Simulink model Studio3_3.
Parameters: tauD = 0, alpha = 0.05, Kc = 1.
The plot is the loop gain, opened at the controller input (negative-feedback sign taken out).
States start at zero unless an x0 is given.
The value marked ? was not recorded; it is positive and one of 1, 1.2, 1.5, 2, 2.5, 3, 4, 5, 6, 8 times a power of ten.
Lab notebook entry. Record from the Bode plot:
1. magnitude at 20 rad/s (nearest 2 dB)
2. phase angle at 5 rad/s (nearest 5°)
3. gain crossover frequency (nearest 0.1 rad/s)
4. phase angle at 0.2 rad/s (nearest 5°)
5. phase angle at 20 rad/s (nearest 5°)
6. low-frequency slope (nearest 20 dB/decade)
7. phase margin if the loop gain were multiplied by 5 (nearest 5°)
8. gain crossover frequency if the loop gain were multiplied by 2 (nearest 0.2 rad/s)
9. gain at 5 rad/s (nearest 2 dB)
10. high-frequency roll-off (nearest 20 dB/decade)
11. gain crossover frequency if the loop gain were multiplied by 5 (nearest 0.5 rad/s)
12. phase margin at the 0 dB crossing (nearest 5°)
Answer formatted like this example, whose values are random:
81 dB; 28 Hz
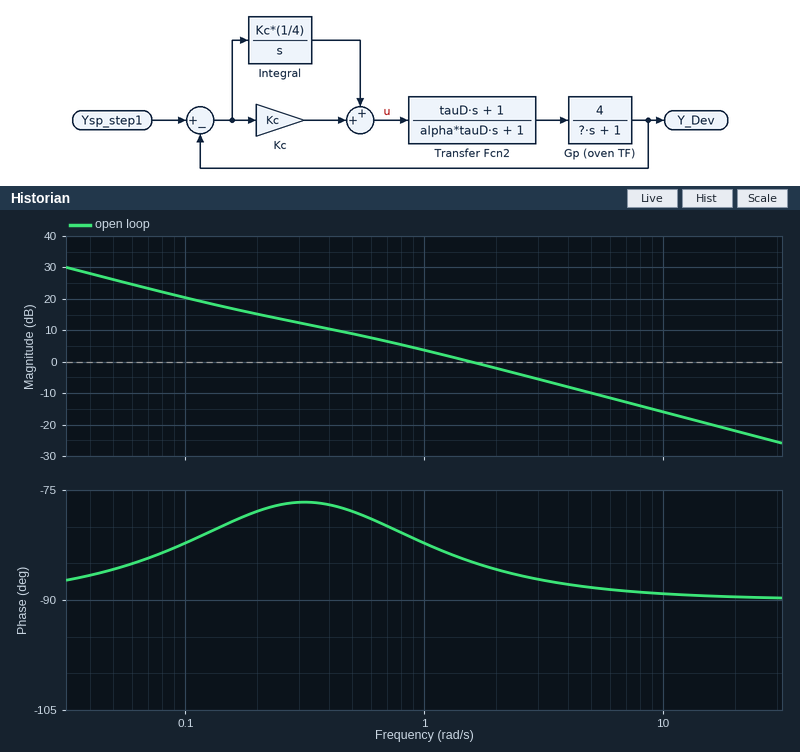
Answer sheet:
-22 dB; -90°; 1.6 rad/s; -80°; -90°; -20 dB/decade; 90°; 3.2 rad/s; -10 dB; -20 dB/decade; 8.0 rad/s; 95°
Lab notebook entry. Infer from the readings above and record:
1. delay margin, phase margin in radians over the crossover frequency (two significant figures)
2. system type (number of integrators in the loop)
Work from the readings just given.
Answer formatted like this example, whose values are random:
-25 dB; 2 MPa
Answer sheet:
1.0 s; 1
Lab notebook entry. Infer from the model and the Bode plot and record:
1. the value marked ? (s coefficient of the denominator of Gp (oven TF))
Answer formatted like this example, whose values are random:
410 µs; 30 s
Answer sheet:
2.5
